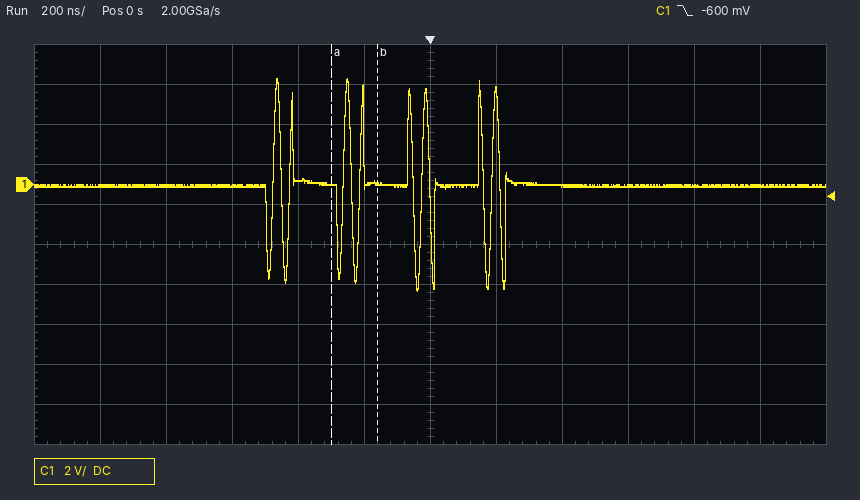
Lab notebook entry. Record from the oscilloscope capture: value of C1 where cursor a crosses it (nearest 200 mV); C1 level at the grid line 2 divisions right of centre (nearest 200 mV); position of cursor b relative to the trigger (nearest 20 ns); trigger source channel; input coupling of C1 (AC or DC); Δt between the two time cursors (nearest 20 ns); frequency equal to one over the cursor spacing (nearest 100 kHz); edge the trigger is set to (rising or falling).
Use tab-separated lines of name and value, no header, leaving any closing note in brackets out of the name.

value of C1 where cursor a crosses it	0.0 V
C1 level at the grid line 2 divisions right of centre	0.0 V
position of cursor b relative to the trigger	-160 ns
trigger source channel	C1
input coupling of C1	DC
Δt between the two time cursors	140 ns
frequency equal to one over the cursor spacing	7.1 MHz
edge the trigger is set to	falling
